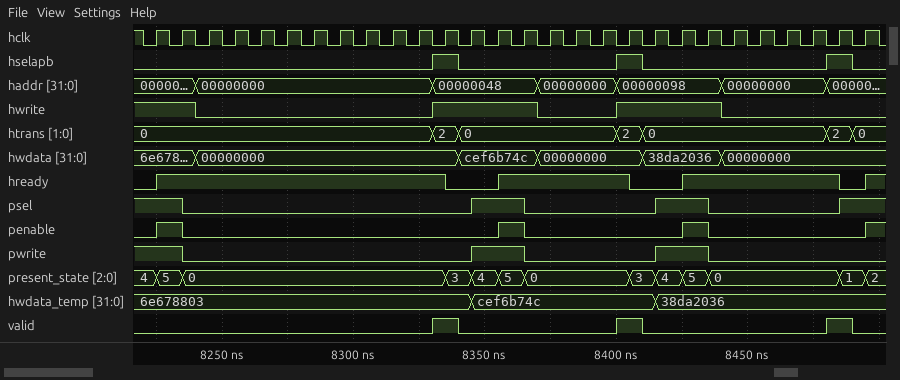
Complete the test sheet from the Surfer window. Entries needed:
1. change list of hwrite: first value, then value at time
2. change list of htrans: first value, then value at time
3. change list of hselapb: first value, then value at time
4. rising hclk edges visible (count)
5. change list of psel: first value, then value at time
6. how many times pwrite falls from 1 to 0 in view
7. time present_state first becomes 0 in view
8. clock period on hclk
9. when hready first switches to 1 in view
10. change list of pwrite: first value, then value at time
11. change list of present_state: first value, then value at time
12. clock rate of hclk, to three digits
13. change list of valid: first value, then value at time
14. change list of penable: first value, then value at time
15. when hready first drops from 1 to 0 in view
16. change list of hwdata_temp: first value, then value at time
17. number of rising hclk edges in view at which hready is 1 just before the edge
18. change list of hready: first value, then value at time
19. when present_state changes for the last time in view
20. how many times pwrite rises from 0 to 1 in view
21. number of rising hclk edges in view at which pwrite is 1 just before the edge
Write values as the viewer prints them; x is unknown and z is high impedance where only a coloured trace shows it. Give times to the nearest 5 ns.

1, 0 at 8240 ns, 1 at 8330 ns, 0 at 8370 ns, 1 at 8400 ns, 0 at 8440 ns
0, 2 at 8330 ns, 0 at 8340 ns, 2 at 8400 ns, 0 at 8410 ns, 2 at 8480 ns, 0 at 8490 ns
0, 1 at 8330 ns, 0 at 8340 ns, 1 at 8400 ns, 0 at 8410 ns, 1 at 8480 ns, 0 at 8490 ns
28
1, 0 at 8235 ns, 1 at 8345 ns, 0 at 8365 ns, 1 at 8415 ns, 0 at 8435 ns, 1 at 8485 ns
3
8235 ns
10 ns
8225 ns
1, 0 at 8235 ns, 1 at 8345 ns, 0 at 8365 ns, 1 at 8415 ns, 0 at 8435 ns
4, 5 at 8225 ns, 0 at 8235 ns, 3 at 8335 ns, 4 at 8345 ns, 5 at 8355 ns, 0 at 8365 ns, 3 at 8405 ns, 4 at 8415 ns, 5 at 8425 ns, 0 at 8435 ns, 1 at 8485 ns, 2 at 8495 ns
100 MHz
0, 1 at 8330 ns, 0 at 8340 ns, 1 at 8400 ns, 0 at 8410 ns, 1 at 8480 ns, 0 at 8490 ns
0, 1 at 8225 ns, 0 at 8235 ns, 1 at 8355 ns, 0 at 8365 ns, 1 at 8425 ns, 0 at 8435 ns, 1 at 8495 ns
8335 ns
6e678803, cef6b74c at 8345 ns, 38da2036 at 8415 ns
22
0, 1 at 8225 ns, 0 at 8335 ns, 1 at 8355 ns, 0 at 8405 ns, 1 at 8425 ns, 0 at 8485 ns, 1 at 8495 ns
8495 ns
2
6
